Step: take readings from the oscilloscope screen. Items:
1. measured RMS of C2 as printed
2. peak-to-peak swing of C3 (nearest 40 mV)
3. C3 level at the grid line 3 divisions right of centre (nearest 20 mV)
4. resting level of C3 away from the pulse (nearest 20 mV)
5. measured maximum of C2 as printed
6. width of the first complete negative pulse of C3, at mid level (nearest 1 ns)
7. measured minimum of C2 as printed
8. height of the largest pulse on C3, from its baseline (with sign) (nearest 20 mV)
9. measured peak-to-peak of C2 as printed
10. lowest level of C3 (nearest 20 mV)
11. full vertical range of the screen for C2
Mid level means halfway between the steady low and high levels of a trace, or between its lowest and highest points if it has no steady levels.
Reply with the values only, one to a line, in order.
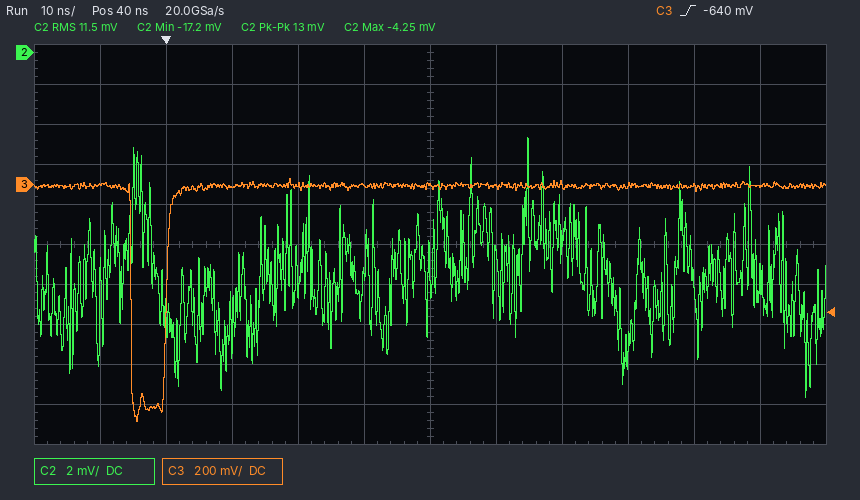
11.5 mV
1.20 V
0 mV
0 mV
-4.25 mV
5 ns
-17.2 mV
-1.18 V
13 mV
-1.18 V
20 mV
